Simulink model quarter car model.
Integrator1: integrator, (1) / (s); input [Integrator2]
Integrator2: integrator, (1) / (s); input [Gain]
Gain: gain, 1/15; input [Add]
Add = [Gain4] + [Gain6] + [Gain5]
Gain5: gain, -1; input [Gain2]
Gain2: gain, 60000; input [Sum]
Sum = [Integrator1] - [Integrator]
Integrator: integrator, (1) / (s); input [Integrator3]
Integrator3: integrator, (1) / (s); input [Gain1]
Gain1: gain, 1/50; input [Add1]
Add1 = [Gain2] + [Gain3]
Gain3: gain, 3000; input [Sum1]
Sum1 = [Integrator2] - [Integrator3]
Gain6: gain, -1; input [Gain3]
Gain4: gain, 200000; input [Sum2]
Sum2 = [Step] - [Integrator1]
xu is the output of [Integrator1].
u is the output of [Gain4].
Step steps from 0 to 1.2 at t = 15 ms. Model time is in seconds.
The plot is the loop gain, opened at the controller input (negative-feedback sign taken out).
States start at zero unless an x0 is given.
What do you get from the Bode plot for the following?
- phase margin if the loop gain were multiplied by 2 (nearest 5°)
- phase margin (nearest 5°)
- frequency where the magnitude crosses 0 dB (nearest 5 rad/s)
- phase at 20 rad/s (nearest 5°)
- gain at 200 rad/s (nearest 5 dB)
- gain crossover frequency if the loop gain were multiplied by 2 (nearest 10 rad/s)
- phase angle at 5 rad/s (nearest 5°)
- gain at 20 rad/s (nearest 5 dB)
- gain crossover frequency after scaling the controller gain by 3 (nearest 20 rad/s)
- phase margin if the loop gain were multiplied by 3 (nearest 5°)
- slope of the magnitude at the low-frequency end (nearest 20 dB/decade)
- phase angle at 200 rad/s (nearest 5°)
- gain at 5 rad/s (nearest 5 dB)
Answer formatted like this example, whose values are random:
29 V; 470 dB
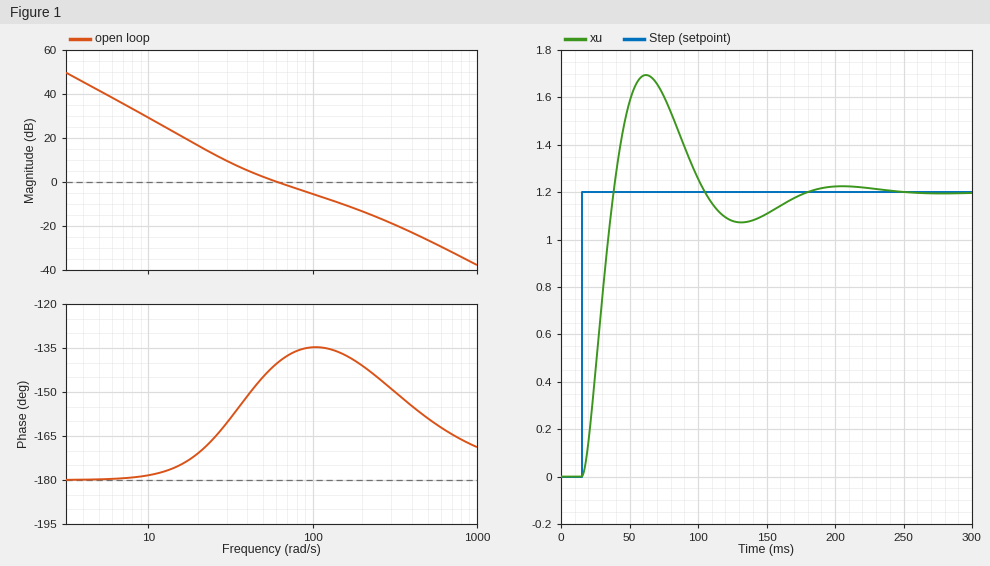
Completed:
45°; 40°; 60 rad/s; -170°; -15 dB; 110 rad/s; -180°; 15 dB; 140 rad/s; 45°; -40 dB/decade; -140°; 40 dB
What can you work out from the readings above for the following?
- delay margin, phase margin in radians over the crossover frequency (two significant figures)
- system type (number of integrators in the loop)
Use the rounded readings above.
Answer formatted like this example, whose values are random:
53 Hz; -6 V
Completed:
0.012 s; 2
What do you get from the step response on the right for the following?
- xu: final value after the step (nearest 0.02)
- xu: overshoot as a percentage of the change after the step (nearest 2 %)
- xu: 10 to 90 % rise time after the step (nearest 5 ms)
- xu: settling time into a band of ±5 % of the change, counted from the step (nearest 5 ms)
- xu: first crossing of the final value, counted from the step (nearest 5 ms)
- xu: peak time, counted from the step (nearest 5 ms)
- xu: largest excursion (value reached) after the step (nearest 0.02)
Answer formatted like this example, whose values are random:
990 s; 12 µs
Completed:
1.20; 42 %; 15 ms; 145 ms; 25 ms; 45 ms; 1.70
